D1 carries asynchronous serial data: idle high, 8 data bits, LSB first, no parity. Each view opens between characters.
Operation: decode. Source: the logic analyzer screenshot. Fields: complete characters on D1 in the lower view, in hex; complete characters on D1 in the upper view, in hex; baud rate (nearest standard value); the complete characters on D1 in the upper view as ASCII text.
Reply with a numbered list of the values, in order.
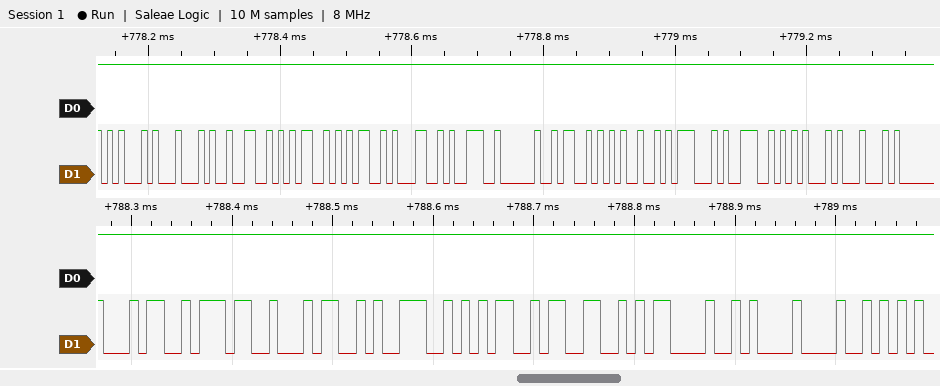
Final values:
1. 34, 37, 34, 39, 35, 33, 0D, 0A, 48
2. 45, 44, 32, 35, 35, 31, 39, 20, 53, 49, 47, 4E, 45, 44
3. 115200 baud
4. "ED25519 SIGNED"
